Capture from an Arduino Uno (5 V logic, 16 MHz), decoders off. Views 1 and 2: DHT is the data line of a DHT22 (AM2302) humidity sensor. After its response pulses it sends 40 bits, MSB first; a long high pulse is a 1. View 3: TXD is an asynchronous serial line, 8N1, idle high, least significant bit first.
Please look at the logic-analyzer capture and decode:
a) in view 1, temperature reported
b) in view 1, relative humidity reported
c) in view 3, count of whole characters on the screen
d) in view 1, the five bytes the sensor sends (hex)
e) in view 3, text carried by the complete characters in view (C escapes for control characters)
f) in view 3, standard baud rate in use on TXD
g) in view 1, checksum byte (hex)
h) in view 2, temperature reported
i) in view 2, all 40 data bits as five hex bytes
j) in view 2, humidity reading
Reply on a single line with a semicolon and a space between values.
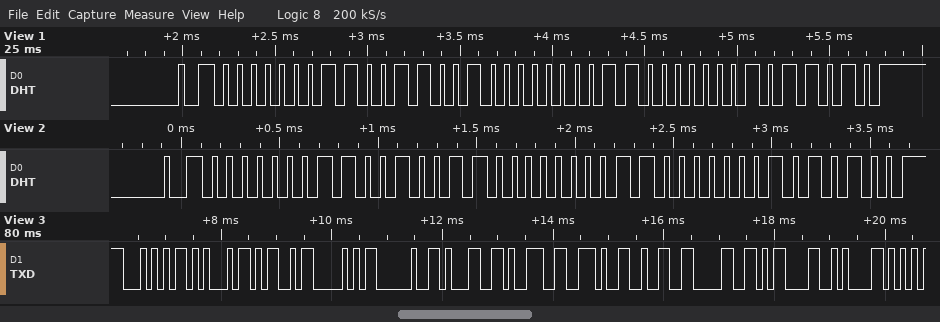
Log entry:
19.2 °C; 40.9 %; 12; 01 99 00 C0 5A; "TEMP 19.20\r\n"; 9600 baud; 0x5A; 19.2 °C; 01 93 00 C0 54; 40.3 %
